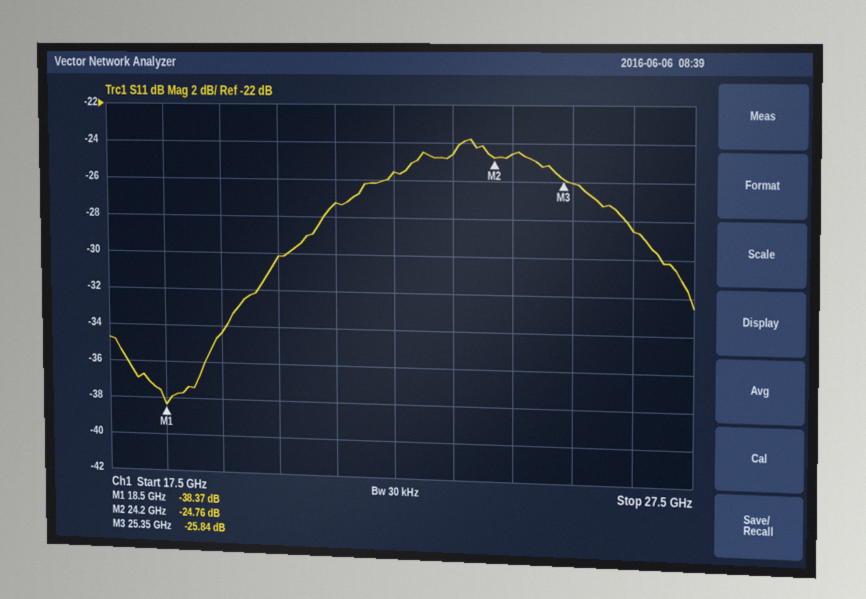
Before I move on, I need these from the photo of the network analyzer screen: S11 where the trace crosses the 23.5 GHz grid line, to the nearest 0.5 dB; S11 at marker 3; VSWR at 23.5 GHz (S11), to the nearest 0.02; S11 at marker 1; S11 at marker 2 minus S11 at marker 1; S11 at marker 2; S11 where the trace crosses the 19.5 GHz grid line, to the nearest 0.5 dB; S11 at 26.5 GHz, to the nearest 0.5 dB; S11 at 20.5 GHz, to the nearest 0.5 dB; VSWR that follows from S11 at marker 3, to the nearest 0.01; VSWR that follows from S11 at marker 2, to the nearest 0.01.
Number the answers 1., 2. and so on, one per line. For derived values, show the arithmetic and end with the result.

1. -24.5 dB
2. -25.84 dB
3. |Γ| = 10^(-24.5/20) = 0.0596; VSWR = (1 + 0.0596)/(1 − 0.0596) ≈ 1.13, so 1.12 to the nearest 0.02
4. -38.37 dB
5. -24.76 − (-38.37) = 13.61 dB
6. -24.76 dB
7. -34.5 dB
8. -28.5 dB
9. -30.0 dB
10. (1 + 0.0511)/(1 − 0.0511) ≈ 1.11
11. (1 + 0.0578)/(1 − 0.0578) ≈ 1.12
